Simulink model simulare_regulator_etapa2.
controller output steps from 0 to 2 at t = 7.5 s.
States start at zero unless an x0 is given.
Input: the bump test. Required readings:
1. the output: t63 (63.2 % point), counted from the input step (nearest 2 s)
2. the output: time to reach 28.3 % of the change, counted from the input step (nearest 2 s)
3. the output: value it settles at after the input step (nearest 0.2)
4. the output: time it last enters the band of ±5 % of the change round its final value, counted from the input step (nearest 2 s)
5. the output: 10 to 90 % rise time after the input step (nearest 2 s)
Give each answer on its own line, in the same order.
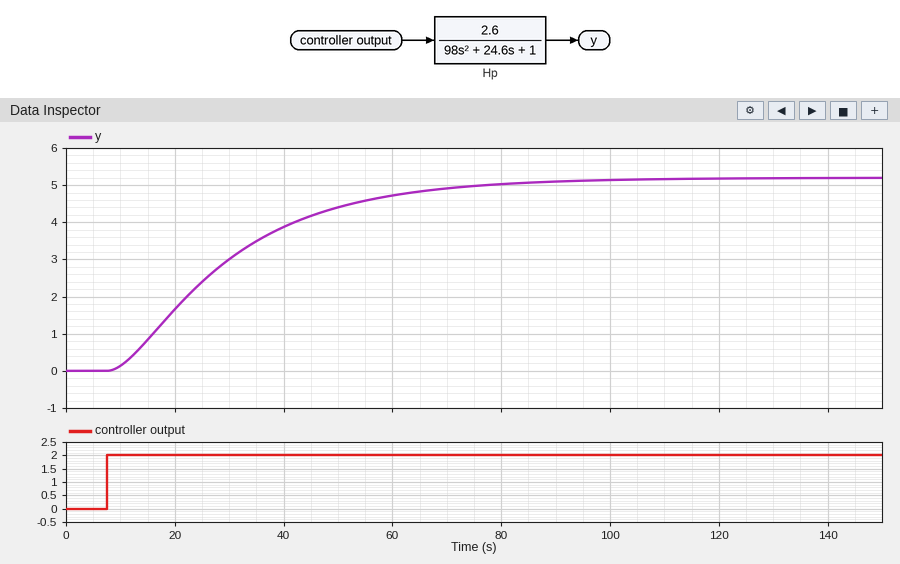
26 s
12 s
5.2
64 s
46 s
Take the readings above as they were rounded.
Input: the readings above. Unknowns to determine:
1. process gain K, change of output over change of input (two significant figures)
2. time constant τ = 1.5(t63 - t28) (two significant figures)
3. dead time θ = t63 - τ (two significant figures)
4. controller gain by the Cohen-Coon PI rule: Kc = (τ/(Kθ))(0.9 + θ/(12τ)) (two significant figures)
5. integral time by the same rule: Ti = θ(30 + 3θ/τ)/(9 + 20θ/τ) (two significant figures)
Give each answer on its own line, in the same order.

2.6
21 s
5.0 s
1.5
11 s
